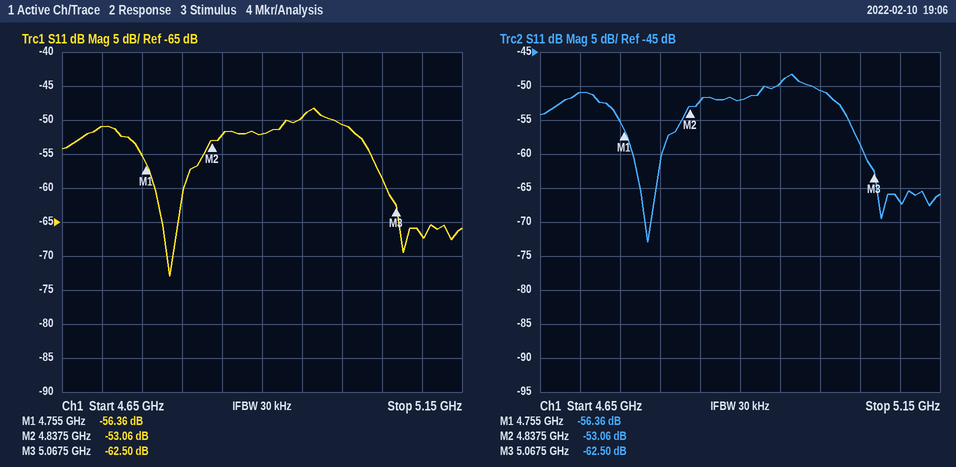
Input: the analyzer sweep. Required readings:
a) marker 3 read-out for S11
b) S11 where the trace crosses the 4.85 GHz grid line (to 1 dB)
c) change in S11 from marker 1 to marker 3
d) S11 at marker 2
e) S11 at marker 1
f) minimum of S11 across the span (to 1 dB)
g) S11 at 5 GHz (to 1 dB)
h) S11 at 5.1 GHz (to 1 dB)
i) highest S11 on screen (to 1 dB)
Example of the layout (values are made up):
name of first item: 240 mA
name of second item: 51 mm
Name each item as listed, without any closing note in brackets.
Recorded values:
marker 3 read-out for S11: -62.50 dB
S11 where the trace crosses the 4.85 GHz grid line: -52 dB
change in S11 from marker 1 to marker 3: -6.14 dB
S11 at marker 2: -53.06 dB
S11 at marker 1: -56.36 dB
minimum of S11 across the span: -73 dB
S11 at 5 GHz: -51 dB
S11 at 5.1 GHz: -67 dB
highest S11 on screen: -48 dB
